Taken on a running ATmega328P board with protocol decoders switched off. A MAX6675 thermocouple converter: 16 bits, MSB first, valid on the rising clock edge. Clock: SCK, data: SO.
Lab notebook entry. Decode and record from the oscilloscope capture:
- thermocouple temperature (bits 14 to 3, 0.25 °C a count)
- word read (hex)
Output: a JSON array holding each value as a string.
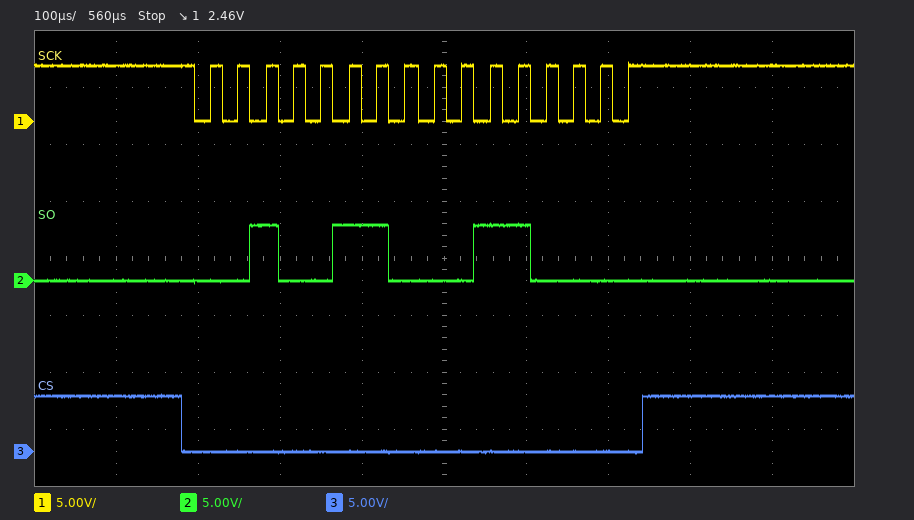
["305.50 °C", "0x2630"]
